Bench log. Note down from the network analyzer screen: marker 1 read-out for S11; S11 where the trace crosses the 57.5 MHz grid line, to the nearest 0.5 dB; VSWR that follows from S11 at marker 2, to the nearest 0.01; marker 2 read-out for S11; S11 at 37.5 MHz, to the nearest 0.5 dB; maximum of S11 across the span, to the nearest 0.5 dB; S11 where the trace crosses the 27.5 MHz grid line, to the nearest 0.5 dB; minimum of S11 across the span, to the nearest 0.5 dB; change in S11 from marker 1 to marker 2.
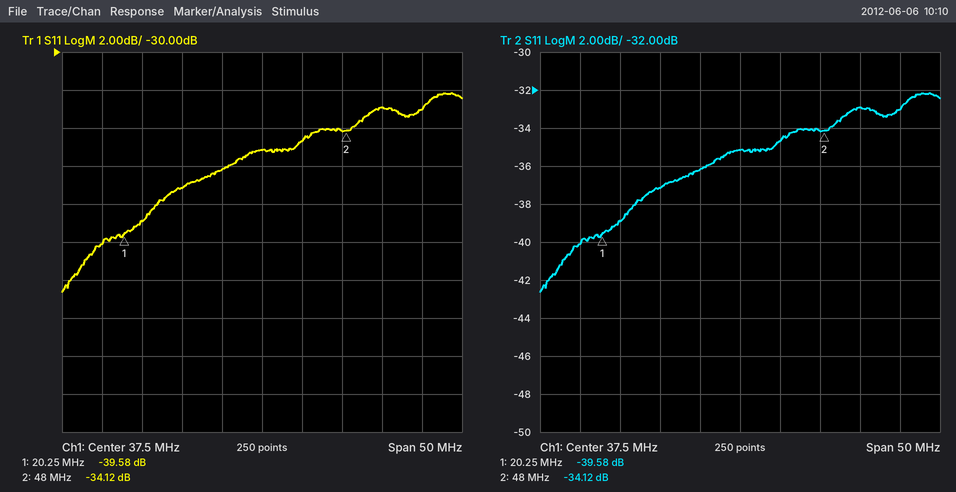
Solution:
-39.58 dB
-33.0 dB
1.04
-34.12 dB
-35.0 dB
-32.0 dB
-37.0 dB
-42.5 dB
5.46 dB
